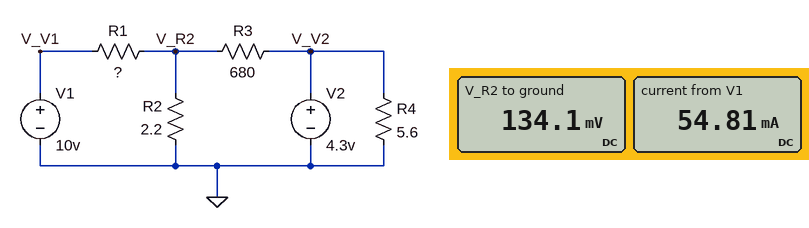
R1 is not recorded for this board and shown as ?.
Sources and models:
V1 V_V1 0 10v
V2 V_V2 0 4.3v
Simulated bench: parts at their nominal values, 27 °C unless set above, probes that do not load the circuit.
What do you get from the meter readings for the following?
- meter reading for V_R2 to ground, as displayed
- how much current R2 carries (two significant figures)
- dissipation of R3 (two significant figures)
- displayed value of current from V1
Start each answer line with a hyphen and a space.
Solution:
- 134.1 mV
- 61 mA
- 26 mW
- 54.81 mA
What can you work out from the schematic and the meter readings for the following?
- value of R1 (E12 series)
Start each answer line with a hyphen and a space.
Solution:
- 180 Ω
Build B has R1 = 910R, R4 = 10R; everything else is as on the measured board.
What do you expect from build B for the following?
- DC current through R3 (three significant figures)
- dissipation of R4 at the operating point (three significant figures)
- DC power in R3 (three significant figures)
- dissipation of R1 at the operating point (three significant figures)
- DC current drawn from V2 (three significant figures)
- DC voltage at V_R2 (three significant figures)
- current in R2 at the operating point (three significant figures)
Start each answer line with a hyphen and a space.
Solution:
- 6.27 mA
- 1.85 W
- 26.7 mW
- 109 mW
- 436 mA
- 37.9 mV
- 17.2 mA
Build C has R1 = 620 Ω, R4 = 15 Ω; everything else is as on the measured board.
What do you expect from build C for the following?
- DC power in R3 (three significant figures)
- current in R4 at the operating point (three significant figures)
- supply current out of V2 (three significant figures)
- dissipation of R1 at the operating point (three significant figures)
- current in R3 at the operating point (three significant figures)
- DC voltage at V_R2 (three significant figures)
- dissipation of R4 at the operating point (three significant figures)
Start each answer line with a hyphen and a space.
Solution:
- 26.6 mW
- 287 mA
- 293 mA
- 160 mW
- 6.25 mA
- 49.1 mV
- 1.23 W
